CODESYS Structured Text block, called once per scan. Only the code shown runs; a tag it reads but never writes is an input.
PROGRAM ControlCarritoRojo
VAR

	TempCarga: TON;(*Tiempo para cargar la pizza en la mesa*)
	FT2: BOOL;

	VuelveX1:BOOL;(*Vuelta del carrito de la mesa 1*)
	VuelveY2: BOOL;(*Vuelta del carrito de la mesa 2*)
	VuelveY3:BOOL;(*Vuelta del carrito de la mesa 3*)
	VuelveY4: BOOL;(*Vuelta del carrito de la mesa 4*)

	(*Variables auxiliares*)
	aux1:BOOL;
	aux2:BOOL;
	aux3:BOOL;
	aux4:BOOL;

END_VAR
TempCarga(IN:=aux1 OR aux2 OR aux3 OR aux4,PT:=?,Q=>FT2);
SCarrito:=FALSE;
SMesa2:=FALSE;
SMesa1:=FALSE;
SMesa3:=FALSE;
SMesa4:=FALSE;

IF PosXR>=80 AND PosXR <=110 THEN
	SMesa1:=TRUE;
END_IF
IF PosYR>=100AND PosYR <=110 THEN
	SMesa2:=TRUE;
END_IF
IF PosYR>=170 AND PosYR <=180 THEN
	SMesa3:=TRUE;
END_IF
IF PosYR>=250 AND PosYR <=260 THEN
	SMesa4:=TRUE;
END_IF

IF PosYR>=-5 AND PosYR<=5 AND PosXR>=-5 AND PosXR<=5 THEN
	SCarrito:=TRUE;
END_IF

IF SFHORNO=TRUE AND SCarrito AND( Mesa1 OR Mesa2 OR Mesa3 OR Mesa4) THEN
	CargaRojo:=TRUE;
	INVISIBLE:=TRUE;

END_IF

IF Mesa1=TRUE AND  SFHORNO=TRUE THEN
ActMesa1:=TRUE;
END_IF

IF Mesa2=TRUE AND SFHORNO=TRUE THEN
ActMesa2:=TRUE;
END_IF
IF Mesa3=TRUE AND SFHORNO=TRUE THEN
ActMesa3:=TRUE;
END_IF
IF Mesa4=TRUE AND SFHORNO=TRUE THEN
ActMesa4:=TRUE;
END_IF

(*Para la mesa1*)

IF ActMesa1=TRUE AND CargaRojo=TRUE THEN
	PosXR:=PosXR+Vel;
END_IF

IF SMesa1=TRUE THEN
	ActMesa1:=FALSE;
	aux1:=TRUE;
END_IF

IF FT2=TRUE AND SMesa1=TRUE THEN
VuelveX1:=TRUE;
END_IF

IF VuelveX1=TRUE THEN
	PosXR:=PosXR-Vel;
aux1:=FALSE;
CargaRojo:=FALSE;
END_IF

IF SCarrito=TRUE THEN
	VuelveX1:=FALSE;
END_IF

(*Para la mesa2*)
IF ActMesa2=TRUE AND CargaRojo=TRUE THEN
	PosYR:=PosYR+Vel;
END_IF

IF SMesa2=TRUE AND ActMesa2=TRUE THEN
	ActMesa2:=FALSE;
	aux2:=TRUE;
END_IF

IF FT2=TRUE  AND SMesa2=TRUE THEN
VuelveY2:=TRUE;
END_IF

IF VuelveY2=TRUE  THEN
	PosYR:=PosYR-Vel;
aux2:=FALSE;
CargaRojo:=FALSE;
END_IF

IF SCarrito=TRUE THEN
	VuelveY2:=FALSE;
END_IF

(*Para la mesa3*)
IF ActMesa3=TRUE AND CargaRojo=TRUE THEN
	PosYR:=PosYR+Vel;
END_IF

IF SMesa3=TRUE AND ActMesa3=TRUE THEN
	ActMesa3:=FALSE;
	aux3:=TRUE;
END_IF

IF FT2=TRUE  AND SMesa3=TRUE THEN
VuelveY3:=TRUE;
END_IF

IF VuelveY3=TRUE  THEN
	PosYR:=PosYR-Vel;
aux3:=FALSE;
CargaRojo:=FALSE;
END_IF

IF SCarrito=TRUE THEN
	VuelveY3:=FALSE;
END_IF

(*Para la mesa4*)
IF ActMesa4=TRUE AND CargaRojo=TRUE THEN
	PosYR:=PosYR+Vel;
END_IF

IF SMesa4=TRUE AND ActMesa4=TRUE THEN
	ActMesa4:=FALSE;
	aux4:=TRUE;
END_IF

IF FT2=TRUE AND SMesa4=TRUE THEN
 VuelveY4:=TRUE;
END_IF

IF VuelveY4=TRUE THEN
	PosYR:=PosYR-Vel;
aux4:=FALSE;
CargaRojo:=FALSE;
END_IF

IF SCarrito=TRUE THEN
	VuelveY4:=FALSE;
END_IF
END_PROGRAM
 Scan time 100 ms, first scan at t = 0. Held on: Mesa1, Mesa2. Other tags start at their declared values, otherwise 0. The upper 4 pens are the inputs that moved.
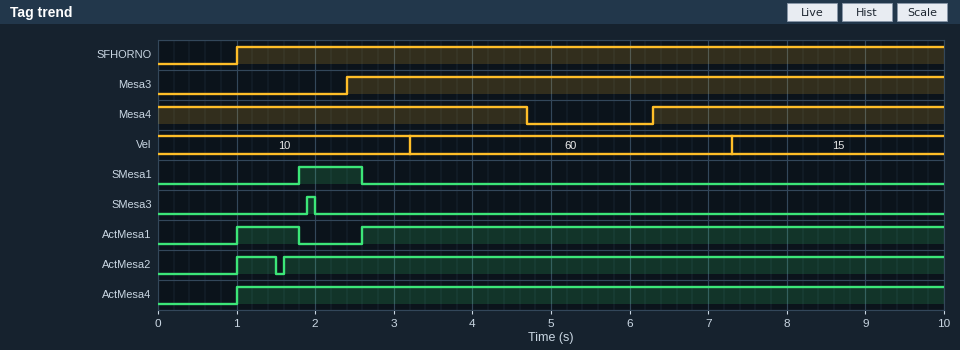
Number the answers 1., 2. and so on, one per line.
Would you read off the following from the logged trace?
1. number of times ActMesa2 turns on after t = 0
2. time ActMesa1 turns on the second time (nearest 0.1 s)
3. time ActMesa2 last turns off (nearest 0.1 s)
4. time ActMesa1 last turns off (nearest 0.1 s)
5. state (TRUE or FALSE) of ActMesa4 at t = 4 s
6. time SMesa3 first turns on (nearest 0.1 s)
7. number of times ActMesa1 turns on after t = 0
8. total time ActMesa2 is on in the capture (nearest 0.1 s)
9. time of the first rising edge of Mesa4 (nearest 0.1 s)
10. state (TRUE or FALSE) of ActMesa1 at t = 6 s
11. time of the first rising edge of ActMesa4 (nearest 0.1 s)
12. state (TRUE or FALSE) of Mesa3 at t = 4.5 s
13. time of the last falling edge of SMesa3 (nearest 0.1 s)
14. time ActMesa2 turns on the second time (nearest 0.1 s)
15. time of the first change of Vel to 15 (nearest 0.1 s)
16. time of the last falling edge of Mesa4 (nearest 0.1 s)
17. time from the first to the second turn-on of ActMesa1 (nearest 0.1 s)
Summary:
1. 2
2. 2.6 s
3. 1.5 s
4. 1.8 s
5. TRUE
6. 1.9 s
7. 2
8. 8.9 s
9. 6.3 s
10. TRUE
11. 1.0 s
12. TRUE
13. 2.0 s
14. 1.6 s
15. 7.3 s
16. 4.7 s
17. 1.6 s
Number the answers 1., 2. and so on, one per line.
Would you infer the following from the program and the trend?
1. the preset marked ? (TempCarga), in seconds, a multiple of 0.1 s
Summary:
1. 0.5 s
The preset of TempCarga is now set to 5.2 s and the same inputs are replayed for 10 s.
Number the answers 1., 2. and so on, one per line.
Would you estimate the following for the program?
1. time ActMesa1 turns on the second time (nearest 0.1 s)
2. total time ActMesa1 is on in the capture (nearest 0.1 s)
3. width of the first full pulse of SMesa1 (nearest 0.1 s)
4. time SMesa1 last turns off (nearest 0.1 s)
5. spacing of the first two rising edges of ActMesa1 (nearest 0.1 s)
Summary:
1. 2.2 s
2. 8.6 s
3. 0.4 s
4. 2.2 s
5. 1.2 s
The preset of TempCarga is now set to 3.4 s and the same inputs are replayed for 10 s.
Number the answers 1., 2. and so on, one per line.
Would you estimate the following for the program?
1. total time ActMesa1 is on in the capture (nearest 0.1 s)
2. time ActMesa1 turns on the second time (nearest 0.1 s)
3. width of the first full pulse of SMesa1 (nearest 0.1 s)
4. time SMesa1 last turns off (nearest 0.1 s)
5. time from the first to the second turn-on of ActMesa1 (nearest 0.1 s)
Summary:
1. 8.6 s
2. 2.2 s
3. 0.4 s
4. 2.2 s
5. 1.2 s
